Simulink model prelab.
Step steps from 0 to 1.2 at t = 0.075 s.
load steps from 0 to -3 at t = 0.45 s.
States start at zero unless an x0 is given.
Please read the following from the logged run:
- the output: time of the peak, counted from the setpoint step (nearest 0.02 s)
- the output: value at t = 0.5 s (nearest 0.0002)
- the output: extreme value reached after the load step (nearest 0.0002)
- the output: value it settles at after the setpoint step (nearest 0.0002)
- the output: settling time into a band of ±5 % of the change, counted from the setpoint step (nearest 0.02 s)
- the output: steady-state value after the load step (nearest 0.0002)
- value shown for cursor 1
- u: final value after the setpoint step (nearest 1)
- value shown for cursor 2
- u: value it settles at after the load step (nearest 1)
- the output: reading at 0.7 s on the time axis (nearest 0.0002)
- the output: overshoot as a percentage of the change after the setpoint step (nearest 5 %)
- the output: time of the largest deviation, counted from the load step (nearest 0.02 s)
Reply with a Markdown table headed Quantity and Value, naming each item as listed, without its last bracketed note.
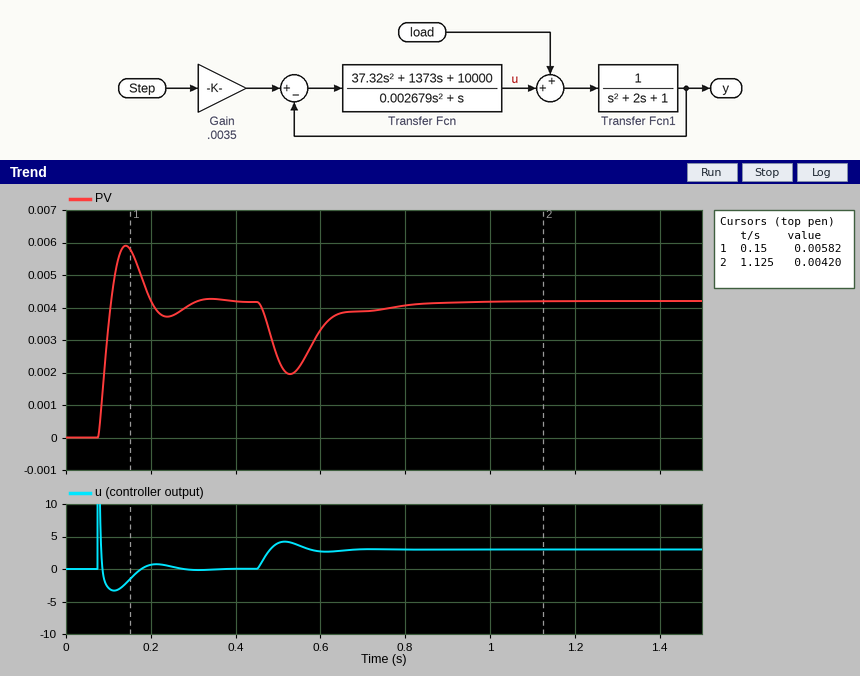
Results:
| Quantity | Value |
|---|---|
| the output: time of the peak, counted from the setpoint step | 0.06 s |
| the output: value at t = 0.5 s | 0.0024 |
| the output: extreme value reached after the load step | 0.0020 |
| the output: value it settles at after the setpoint step | 0.0042 |
| the output: settling time into a band of ±5 % of the change, counted from the setpoint step | 0.20 s |
| the output: steady-state value after the load step | 0.0042 |
| value shown for cursor 1 | 0.00582 |
| u: final value after the setpoint step | 0 |
| value shown for cursor 2 | 0.00420 |
| u: value it settles at after the load step | 3 |
| the output: reading at 0.7 s on the time axis | 0.0038 |
| the output: overshoot as a percentage of the change after the setpoint step | 40 % |
| the output: time of the largest deviation, counted from the load step | 0.08 s |
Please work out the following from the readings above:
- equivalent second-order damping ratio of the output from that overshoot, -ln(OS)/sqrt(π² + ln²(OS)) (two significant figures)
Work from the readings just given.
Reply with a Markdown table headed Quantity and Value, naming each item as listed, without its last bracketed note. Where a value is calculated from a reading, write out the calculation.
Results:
| Quantity | Value |
|---|---|
| equivalent second-order damping ratio of the output from that overshoot, -ln(OS)/sqrt(π² + ln²(OS)) | ln(0.4) = -0.916; 0.916 / sqrt(9.870 + 0.840) = 0.28 |
